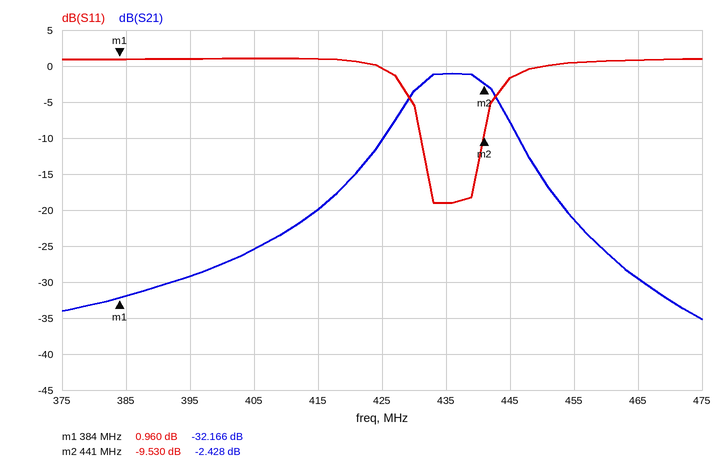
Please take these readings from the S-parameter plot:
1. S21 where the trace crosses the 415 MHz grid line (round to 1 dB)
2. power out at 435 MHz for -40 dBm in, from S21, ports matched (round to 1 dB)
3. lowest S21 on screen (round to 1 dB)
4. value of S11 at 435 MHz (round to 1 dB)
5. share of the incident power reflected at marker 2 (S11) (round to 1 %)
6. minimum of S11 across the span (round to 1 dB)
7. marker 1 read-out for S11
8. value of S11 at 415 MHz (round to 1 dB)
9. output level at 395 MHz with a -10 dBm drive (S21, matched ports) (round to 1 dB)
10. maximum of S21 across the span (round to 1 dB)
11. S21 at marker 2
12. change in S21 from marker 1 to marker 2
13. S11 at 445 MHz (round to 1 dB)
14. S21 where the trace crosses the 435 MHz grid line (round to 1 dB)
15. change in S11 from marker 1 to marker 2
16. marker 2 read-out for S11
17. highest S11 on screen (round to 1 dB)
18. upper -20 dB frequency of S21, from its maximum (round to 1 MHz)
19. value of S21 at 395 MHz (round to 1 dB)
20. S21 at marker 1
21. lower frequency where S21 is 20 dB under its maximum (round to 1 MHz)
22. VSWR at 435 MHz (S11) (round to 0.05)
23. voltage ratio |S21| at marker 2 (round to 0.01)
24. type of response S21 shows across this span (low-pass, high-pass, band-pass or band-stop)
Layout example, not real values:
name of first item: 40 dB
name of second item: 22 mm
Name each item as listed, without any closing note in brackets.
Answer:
S21 where the trace crosses the 415 MHz grid line: -20 dB
power out at 435 MHz for -40 dBm in, from S21, ports matched: -41 dBm
lowest S21 on screen: -35 dB
value of S11 at 435 MHz: -19 dB
share of the incident power reflected at marker 2 (S11): 11 %
minimum of S11 across the span: -19 dB
marker 1 read-out for S11: 0.960 dB
value of S11 at 415 MHz: 1 dB
output level at 395 MHz with a -10 dBm drive (S21, matched ports): -39 dBm
maximum of S21 across the span: -1 dB
S21 at marker 2: -2.428 dB
change in S21 from marker 1 to marker 2: 29.738 dB
S11 at 445 MHz: -2 dB
S21 where the trace crosses the 435 MHz grid line: -1 dB
change in S11 from marker 1 to marker 2: -10.490 dB
marker 2 read-out for S11: -9.530 dB
highest S11 on screen: 1 dB
upper -20 dB frequency of S21, from its maximum: 455 MHz
value of S21 at 395 MHz: -29 dB
S21 at marker 1: -32.166 dB
lower frequency where S21 is 20 dB under its maximum: 413 MHz
VSWR at 435 MHz (S11): 1.25
voltage ratio |S21| at marker 2: 0.76
type of response S21 shows across this span: band-pass
